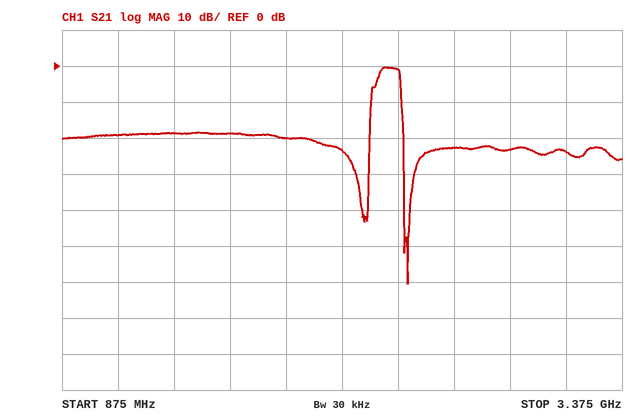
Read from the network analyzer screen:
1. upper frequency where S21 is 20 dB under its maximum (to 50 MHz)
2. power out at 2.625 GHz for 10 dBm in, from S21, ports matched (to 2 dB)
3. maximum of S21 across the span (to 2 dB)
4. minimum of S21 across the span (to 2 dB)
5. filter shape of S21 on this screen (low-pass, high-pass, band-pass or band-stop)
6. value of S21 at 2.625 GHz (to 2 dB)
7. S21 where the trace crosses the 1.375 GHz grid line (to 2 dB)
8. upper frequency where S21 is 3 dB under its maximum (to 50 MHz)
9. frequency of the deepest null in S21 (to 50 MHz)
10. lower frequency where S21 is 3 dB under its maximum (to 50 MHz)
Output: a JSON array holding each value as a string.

["2.40 GHz", "-12 dBm", "0 dB", "-60 dB", "band-pass", "-22 dB", "-18 dB", "2.40 GHz", "2.40 GHz", "2.30 GHz"]
